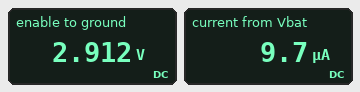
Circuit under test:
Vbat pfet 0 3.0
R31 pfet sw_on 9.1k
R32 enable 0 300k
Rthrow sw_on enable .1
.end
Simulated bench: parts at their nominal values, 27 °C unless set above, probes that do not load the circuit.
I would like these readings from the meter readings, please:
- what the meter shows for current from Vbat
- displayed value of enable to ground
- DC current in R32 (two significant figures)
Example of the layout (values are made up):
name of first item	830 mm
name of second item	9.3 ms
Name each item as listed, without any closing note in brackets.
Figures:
what the meter shows for current from Vbat	9.7 µA
displayed value of enable to ground	2.912 V
DC current in R32	9.7 µA
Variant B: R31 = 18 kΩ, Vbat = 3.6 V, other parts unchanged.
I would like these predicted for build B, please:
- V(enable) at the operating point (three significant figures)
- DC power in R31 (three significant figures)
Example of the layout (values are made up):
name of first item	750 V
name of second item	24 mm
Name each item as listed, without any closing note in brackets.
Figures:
V(enable) at the operating point	3.40 V
DC power in R31	2.31 µW
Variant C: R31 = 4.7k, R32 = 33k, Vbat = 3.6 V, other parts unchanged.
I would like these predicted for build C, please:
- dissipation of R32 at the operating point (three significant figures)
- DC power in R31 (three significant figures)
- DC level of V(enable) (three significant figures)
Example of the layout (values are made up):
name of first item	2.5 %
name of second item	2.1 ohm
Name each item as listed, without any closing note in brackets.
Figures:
dissipation of R32 at the operating point	301 µW
DC power in R31	42.9 µW
DC level of V(enable)	3.15 V
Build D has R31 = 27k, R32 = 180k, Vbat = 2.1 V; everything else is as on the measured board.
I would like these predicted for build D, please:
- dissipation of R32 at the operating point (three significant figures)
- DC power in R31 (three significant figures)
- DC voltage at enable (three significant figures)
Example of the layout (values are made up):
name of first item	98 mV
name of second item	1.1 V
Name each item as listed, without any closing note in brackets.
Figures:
dissipation of R32 at the operating point	18.5 µW
DC power in R31	2.78 µW
DC voltage at enable	1.83 V
